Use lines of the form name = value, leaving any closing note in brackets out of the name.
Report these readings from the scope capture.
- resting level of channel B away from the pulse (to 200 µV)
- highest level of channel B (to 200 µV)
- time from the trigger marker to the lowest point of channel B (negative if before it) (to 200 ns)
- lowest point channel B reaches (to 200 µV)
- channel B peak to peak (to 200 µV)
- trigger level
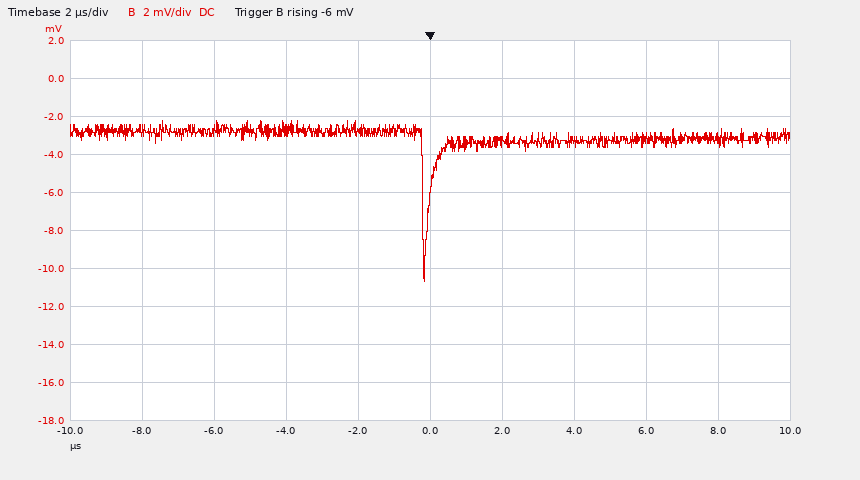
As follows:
resting level of channel B away from the pulse = -3.0 mV
highest level of channel B = -2.2 mV
time from the trigger marker to the lowest point of channel B (negative if before it) = -200 ns
lowest point channel B reaches = -10.6 mV
channel B peak to peak = 8.4 mV
trigger level = -6 mV
